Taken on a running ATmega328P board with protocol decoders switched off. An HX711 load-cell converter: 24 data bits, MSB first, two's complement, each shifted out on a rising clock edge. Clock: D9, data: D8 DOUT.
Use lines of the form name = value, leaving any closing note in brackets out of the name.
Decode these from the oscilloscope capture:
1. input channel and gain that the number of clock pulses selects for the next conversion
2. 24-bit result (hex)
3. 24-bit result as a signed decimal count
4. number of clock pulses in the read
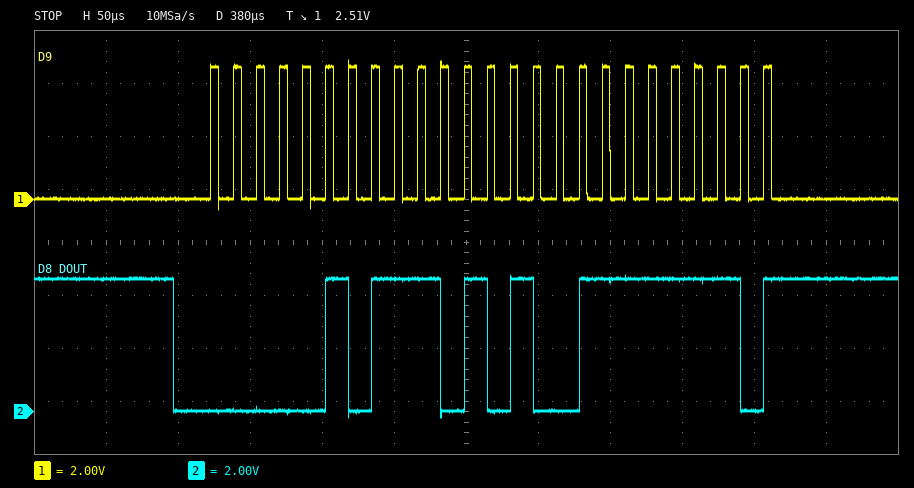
input channel and gain that the number of clock pulses selects for the next conversion = channel A, gain 128
24-bit result = 0x05D4FE
24-bit result as a signed decimal count = 382206
number of clock pulses in the read = 25
